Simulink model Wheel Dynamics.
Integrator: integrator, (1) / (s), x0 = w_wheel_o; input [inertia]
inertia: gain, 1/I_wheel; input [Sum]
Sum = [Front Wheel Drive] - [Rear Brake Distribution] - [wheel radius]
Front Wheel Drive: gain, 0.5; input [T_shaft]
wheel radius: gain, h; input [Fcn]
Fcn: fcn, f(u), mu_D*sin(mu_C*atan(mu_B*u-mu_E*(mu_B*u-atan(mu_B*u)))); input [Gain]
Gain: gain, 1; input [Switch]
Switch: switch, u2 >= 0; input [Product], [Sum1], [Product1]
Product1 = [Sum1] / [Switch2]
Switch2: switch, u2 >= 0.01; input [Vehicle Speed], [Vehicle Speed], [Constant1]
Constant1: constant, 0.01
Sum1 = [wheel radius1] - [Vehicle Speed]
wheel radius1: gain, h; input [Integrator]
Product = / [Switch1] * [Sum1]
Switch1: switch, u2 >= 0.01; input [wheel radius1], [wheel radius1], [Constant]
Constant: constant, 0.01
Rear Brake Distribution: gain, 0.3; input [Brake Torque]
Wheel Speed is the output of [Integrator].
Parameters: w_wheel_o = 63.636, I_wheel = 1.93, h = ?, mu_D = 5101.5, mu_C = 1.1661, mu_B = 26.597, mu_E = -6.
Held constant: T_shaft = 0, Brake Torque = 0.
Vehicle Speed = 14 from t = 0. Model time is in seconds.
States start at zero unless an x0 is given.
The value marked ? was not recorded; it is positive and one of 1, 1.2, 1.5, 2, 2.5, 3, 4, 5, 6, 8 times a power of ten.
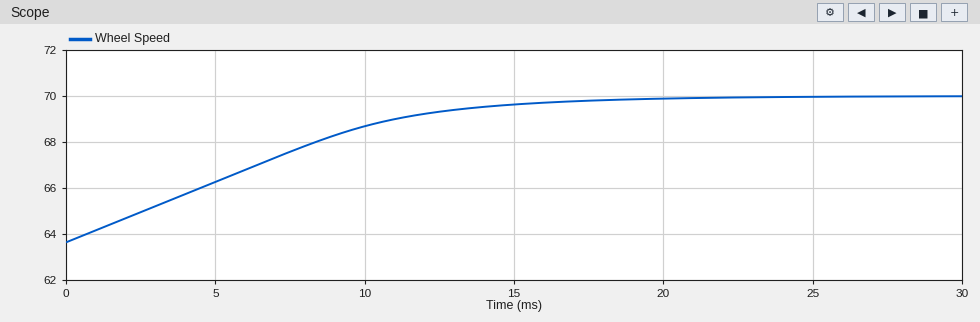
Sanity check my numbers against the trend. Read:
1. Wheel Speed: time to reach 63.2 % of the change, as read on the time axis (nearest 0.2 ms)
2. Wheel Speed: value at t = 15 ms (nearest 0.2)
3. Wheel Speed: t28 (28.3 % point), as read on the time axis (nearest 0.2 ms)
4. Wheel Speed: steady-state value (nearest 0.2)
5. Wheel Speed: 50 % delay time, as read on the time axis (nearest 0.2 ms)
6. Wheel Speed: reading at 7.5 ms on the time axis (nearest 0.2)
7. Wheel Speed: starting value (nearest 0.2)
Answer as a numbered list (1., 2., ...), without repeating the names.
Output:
1. 7.6 ms
2. 69.6
3. 3.4 ms
4. 70.0
5. 6.0 ms
6. 67.6
7. 63.6
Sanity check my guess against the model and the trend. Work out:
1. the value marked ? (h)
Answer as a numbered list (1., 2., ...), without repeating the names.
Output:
1. 0.2
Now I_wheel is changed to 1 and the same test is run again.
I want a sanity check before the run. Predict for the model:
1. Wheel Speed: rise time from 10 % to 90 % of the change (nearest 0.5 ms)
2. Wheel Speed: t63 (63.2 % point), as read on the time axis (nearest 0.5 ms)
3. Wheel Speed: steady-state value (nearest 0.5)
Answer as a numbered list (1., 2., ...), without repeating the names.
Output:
1. 6.0 ms
2. 4.0 ms
3. 70.0
